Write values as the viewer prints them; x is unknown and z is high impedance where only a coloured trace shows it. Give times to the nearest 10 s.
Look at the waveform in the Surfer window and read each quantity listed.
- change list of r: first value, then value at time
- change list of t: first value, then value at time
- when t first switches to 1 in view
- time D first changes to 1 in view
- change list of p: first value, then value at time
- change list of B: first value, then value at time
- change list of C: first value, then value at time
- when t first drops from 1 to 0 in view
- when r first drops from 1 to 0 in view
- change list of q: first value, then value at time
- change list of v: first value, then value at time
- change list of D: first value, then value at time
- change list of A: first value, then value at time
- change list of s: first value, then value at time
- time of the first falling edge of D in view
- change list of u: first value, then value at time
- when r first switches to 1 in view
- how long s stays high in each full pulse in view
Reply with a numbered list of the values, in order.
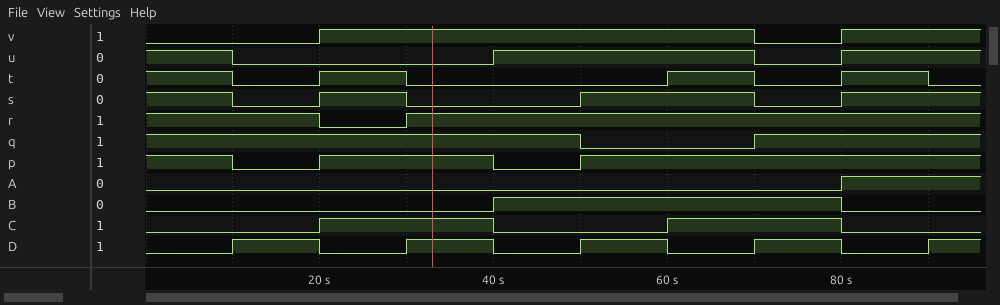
1. 1, 0 at 20 s, 1 at 30 s
2. 1, 0 at 10 s, 1 at 20 s, 0 at 30 s, 1 at 60 s, 0 at 70 s, 1 at 80 s, 0 at 90 s
3. 20 s
4. 10 s
5. 1, 0 at 10 s, 1 at 20 s, 0 at 40 s, 1 at 50 s
6. 0, 1 at 40 s, 0 at 80 s
7. 0, 1 at 20 s, 0 at 40 s, 1 at 60 s, 0 at 80 s
8. 10 s
9. 20 s
10. 1, 0 at 50 s, 1 at 70 s
11. 0, 1 at 20 s, 0 at 70 s, 1 at 80 s
12. 0, 1 at 10 s, 0 at 20 s, 1 at 30 s, 0 at 40 s, 1 at 50 s, 0 at 60 s, 1 at 70 s, 0 at 80 s, 1 at 90 s
13. 0, 1 at 80 s
14. 1, 0 at 10 s, 1 at 20 s, 0 at 30 s, 1 at 50 s, 0 at 70 s, 1 at 80 s
15. 20 s
16. 1, 0 at 10 s, 1 at 40 s, 0 at 70 s, 1 at 80 s
17. 30 s
18. 10 s, 20 s
